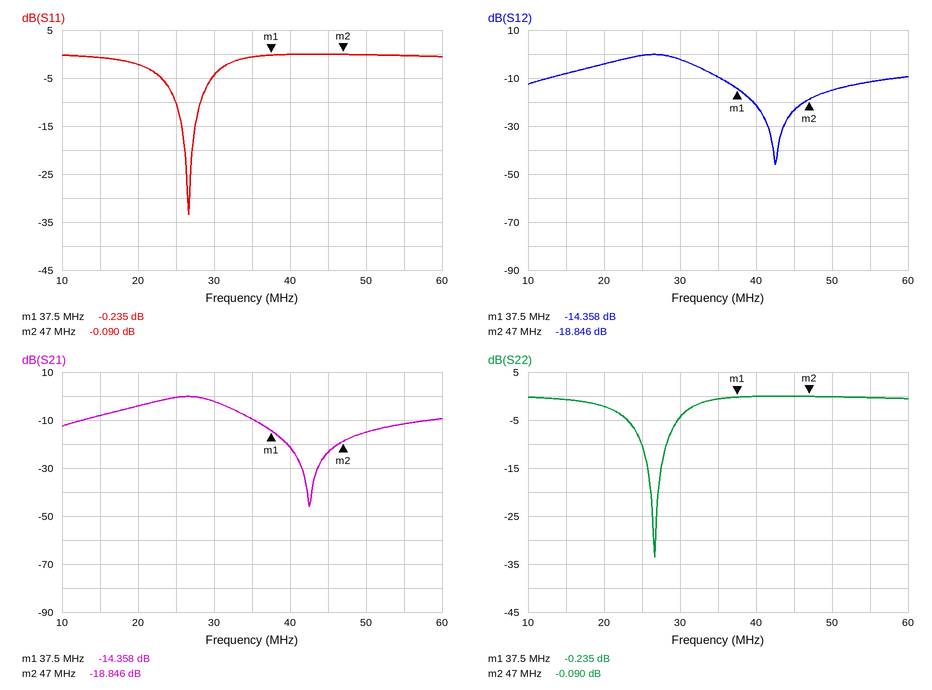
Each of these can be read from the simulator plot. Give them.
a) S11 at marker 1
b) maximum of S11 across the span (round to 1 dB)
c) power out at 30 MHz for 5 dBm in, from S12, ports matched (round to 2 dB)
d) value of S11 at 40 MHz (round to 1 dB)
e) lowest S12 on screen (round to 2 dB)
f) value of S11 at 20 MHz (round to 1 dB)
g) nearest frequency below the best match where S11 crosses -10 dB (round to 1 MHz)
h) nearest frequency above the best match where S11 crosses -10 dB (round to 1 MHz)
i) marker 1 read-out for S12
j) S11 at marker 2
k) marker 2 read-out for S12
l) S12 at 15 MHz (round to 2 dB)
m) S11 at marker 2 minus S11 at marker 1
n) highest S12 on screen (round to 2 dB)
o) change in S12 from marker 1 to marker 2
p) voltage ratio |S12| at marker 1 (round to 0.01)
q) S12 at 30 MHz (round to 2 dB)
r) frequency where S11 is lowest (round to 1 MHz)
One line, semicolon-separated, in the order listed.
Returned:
-0.235 dB; 0 dB; 2 dBm; 0 dB; -46 dB; -2 dB; 25 MHz; 28 MHz; -14.358 dB; -0.090 dB; -18.846 dB; -8 dB; 0.145 dB; 0 dB; -4.488 dB; 0.19; -2 dB; 27 MHz
